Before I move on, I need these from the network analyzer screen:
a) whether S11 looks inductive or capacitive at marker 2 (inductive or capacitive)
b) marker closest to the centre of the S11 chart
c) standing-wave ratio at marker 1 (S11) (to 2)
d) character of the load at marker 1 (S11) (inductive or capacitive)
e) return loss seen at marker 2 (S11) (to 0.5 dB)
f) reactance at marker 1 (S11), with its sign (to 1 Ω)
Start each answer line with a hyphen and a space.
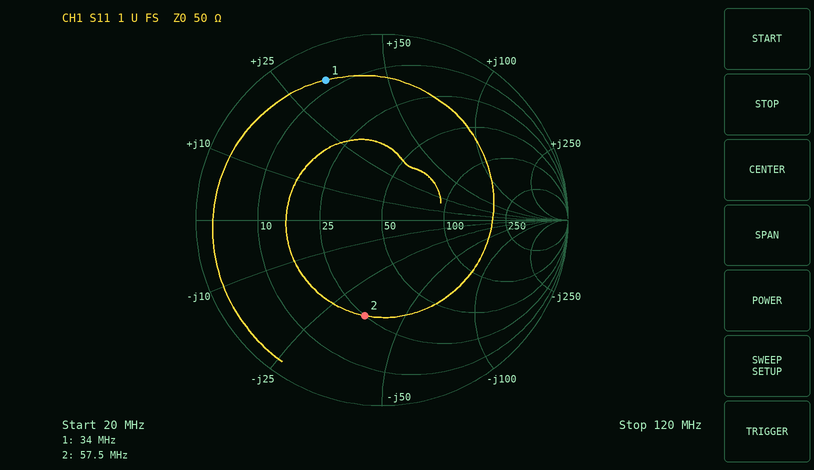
- capacitive
- marker 2
- 10
- inductive
- 5.5 dB
- +33 Ω
